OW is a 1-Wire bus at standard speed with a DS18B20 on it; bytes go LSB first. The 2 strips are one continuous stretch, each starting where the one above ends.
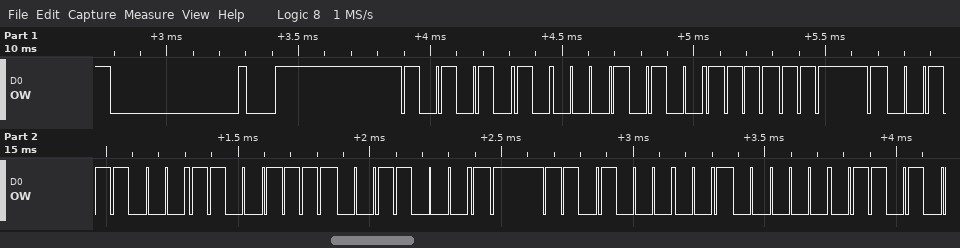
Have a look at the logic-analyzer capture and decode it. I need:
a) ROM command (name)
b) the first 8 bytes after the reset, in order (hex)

Match ROM
55 28 FF 1C F3 8C 17 04
